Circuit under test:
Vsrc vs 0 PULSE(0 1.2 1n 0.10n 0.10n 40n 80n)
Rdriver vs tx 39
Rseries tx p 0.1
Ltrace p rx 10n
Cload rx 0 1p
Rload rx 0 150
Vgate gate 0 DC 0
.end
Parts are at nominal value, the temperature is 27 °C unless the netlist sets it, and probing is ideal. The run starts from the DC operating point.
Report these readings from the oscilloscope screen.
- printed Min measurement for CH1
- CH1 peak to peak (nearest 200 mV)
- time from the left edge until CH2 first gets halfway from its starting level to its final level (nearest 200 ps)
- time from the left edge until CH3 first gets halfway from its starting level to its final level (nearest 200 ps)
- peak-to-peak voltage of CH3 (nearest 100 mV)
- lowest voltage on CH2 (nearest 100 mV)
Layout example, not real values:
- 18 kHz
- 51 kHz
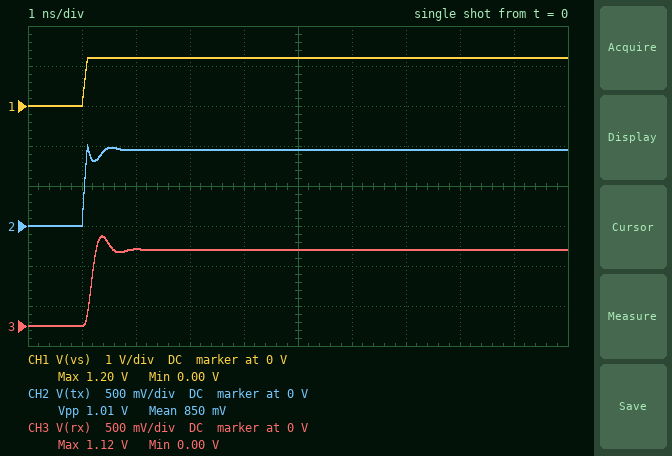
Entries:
- 0.00 V
- 1.2 V
- 1.0 ns
- 1.2 ns
- 1.1 V
- 0 V
